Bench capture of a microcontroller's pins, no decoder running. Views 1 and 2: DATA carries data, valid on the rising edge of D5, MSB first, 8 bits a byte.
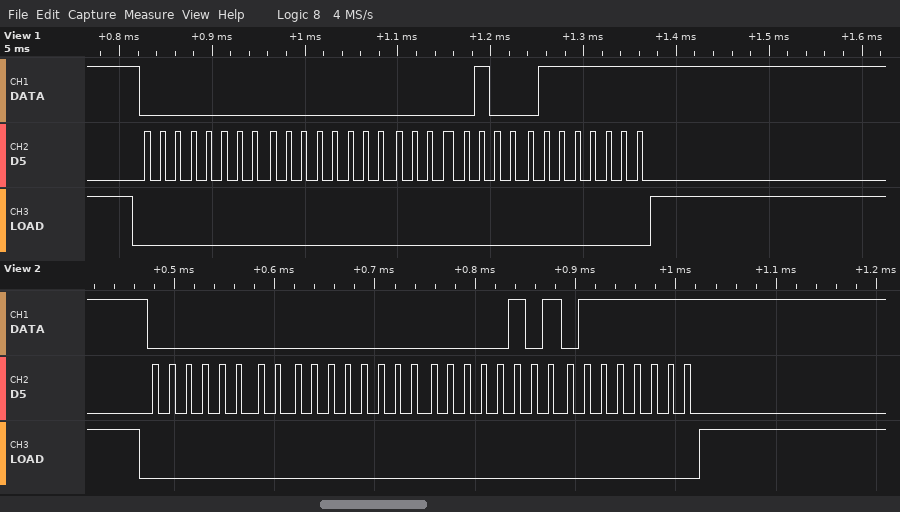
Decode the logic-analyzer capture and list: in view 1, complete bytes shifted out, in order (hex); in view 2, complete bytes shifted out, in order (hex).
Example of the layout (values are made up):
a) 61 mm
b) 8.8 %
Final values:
a) 00 00 04 7F
b) 00 00 05 7F
